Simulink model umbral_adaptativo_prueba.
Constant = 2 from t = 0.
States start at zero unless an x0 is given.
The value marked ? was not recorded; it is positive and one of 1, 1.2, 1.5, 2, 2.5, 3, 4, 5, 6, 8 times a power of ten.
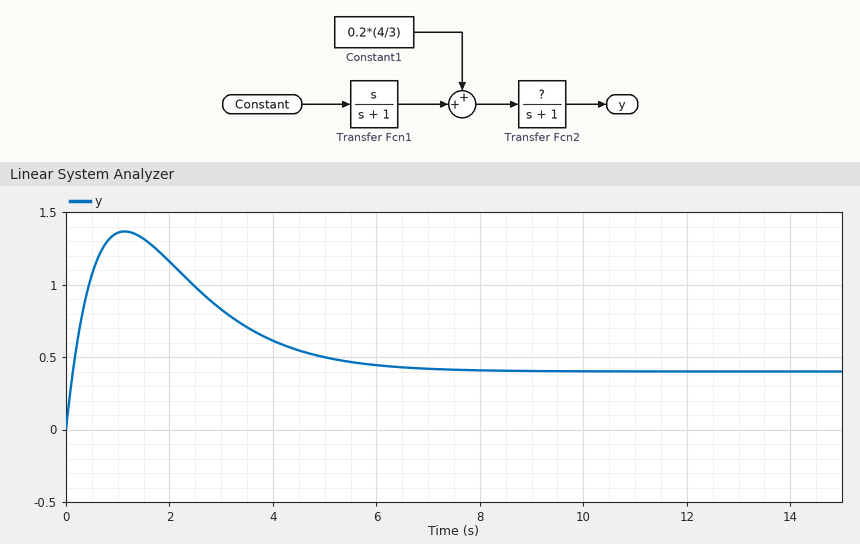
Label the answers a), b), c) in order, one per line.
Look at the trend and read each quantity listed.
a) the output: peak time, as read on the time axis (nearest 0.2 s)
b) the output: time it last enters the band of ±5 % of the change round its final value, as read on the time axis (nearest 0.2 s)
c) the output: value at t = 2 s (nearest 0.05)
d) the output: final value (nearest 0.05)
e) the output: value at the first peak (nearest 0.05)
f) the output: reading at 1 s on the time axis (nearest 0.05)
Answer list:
a) 1.2 s
b) 7.0 s
c) 1.15
d) 0.40
e) 1.35
f) 1.35
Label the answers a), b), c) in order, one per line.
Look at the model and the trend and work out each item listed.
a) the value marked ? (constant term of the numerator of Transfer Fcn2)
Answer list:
a) 1.5
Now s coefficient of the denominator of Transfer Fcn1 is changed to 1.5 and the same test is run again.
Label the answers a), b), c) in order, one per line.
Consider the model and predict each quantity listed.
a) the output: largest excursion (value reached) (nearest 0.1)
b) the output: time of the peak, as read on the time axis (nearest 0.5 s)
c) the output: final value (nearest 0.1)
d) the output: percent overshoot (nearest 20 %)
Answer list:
a) 1.2
b) 1.5 s
c) 0.4
d) 200 %
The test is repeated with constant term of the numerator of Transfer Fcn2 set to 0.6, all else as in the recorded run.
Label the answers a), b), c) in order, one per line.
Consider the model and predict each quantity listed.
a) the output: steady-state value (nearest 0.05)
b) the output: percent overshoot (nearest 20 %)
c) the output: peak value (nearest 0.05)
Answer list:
a) 0.15
b) 240 %
c) 0.55
